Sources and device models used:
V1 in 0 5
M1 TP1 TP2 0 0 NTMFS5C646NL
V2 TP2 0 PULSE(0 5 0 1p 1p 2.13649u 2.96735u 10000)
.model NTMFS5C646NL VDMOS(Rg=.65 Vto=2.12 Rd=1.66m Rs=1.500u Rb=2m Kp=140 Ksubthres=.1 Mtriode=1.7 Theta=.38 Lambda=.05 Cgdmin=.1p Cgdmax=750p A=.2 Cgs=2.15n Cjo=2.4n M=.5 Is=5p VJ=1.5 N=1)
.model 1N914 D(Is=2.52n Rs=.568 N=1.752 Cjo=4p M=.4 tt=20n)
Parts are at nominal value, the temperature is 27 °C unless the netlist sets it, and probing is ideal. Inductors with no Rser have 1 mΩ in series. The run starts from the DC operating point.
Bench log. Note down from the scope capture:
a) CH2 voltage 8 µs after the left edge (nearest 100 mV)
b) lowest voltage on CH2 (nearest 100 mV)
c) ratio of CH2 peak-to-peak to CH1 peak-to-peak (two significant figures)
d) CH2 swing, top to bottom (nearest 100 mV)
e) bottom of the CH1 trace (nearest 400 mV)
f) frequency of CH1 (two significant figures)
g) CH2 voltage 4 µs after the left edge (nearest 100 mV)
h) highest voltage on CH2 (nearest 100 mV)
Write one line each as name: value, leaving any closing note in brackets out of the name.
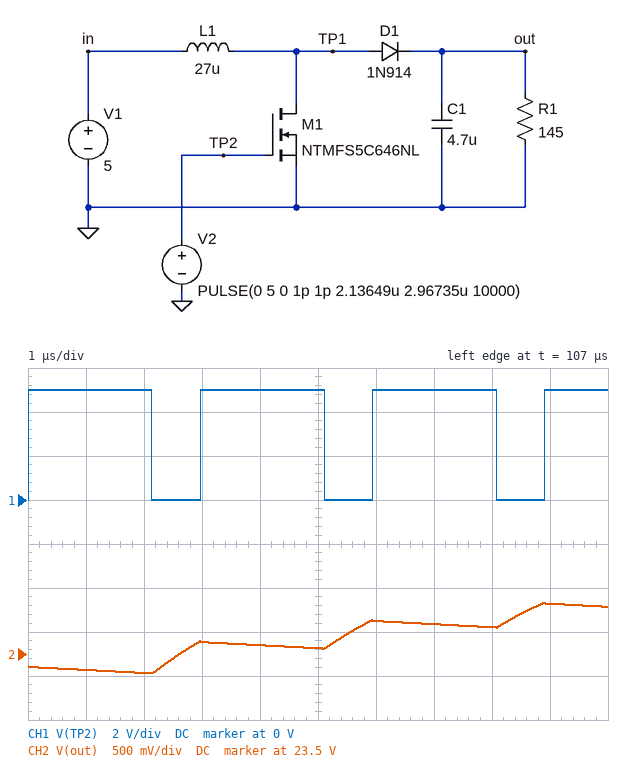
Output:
CH2 voltage 8 µs after the left edge: 23.8 V
lowest voltage on CH2: 23.3 V
ratio of CH2 peak-to-peak to CH1 peak-to-peak: 0.16
CH2 swing, top to bottom: 800 mV
bottom of the CH1 trace: 0 V
frequency of CH1: 340 kHz
CH2 voltage 4 µs after the left edge: 23.6 V
highest voltage on CH2: 24.1 V
